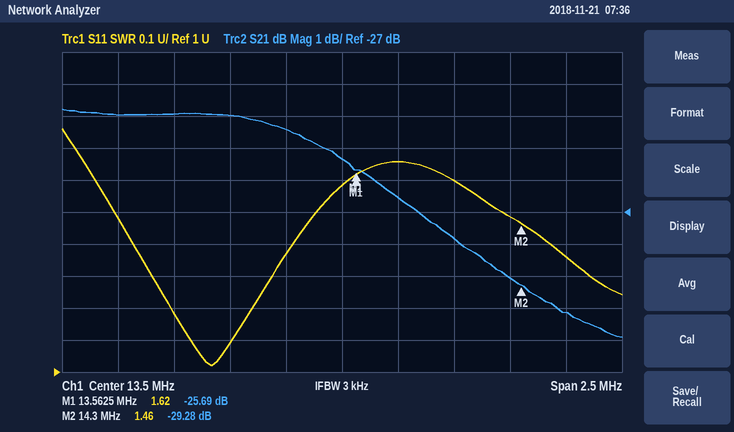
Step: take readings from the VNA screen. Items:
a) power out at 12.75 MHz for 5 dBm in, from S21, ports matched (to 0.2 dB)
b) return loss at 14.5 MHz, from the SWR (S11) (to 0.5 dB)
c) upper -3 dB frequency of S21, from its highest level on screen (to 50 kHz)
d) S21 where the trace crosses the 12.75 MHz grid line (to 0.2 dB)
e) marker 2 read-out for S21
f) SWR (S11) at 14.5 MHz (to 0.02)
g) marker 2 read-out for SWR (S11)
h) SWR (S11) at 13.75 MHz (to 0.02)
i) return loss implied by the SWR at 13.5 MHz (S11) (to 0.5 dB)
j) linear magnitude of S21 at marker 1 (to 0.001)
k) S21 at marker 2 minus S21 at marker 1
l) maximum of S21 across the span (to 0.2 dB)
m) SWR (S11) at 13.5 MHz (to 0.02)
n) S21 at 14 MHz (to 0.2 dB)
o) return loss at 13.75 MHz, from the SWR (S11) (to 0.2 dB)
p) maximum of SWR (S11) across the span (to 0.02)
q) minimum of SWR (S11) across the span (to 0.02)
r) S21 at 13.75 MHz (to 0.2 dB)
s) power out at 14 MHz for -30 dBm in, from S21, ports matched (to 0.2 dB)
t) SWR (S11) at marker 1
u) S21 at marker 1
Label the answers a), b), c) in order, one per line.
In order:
a) -19.0 dBm
b) 16.5 dB
c) 13.80 MHz
d) -24.0 dB
e) -29.28 dB
f) 1.36
g) 1.46
h) 1.66
i) 13.0 dB
j) 0.052
k) -3.59 dB
l) -23.8 dB
m) 1.58
n) -27.8 dB
o) 12.2 dB
p) 1.76
q) 1.02
r) -26.6 dB
s) -57.8 dBm
t) 1.62
u) -25.69 dB
